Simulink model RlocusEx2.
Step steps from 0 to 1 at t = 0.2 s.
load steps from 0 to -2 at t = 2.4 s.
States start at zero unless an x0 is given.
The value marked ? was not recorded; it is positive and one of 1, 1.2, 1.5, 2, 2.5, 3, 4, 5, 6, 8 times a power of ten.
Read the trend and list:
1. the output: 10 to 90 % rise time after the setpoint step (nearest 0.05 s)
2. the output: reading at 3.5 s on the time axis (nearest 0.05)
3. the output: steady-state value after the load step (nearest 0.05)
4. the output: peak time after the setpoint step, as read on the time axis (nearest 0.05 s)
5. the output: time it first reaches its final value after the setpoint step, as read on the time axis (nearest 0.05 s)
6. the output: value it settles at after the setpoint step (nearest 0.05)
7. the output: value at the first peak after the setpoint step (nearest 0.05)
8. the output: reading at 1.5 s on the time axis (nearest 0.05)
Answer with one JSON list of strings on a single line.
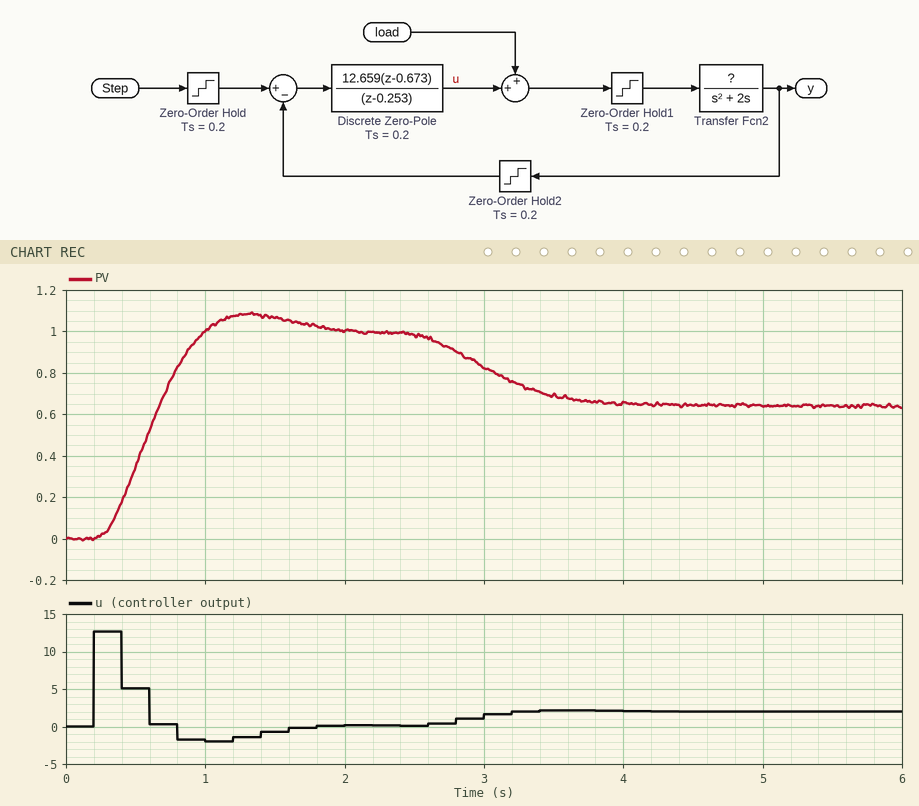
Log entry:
["0.50 s", "0.70", "0.65", "1.30 s", "1.00 s", "1.00", "1.10", "1.05"]
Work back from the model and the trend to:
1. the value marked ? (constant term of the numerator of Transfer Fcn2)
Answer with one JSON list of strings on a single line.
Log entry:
["0.8"]
